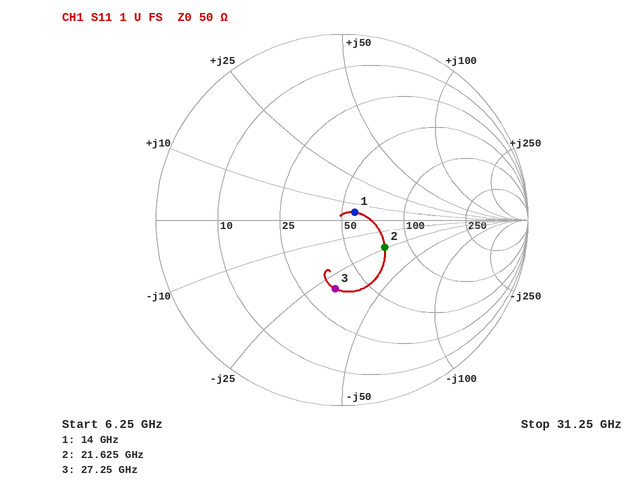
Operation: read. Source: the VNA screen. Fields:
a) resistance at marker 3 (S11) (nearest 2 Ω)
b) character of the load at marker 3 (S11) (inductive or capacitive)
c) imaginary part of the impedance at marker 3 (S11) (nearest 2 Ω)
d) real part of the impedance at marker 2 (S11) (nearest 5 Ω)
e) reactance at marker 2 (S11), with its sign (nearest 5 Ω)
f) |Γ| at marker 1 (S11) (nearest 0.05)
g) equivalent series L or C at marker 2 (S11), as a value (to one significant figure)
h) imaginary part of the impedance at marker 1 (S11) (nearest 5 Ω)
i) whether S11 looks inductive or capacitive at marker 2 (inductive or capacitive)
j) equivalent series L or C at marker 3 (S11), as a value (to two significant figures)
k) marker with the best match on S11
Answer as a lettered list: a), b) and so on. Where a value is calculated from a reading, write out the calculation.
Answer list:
a) 36 Ω
b) capacitive
c) -30 Ω
d) 75 Ω
e) -25 Ω
f) 0.10
g) C = 1/(2π × 21.625 GHz × 25 Ω) ≈ 294 fF, so 300 fF to one significant figure
h) +5 Ω
i) capacitive
j) C = 1/(2π × 27.25 GHz × 30 Ω) ≈ 195 fF, so 190 fF to two significant figures
k) marker 1
